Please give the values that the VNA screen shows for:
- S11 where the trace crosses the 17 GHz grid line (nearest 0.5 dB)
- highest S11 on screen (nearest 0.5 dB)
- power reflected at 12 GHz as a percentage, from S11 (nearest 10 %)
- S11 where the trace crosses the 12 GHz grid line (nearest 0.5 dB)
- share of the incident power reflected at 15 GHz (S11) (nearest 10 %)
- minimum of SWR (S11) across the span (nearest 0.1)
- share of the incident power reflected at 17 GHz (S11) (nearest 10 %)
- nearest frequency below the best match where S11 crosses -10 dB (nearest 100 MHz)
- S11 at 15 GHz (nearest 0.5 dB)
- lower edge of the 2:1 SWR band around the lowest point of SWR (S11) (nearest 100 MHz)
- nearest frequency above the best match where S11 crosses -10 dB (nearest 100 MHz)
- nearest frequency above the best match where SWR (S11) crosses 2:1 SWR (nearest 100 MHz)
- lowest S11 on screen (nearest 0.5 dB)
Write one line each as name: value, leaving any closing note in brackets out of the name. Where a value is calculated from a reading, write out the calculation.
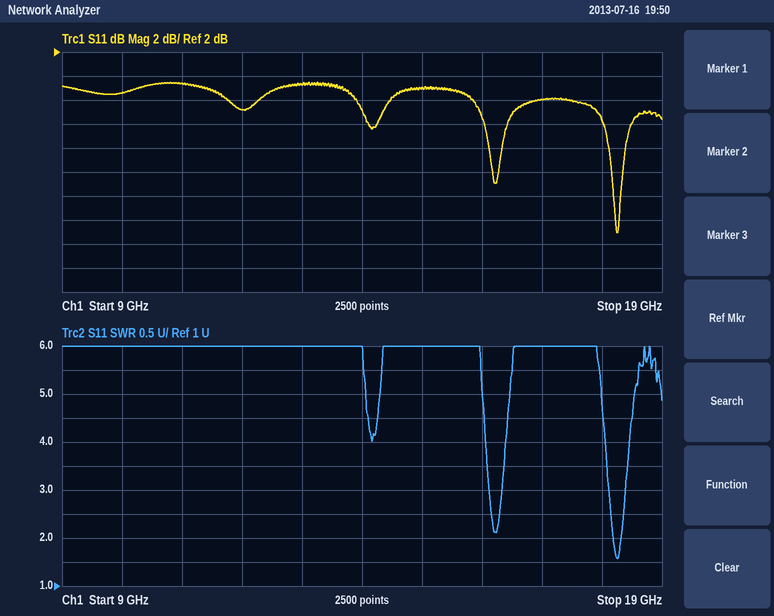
S11 where the trace crosses the 17 GHz grid line: -2.0 dB
highest S11 on screen: -0.5 dB
power reflected at 12 GHz as a percentage, from S11: 10^(-3/10) ≈ 50 %
S11 where the trace crosses the 12 GHz grid line: -3.0 dB
share of the incident power reflected at 15 GHz (S11): 10^(-1/10) ≈ 79.4 %, so 80 % to the nearest 10 %
minimum of SWR (S11) across the span: 1.6
share of the incident power reflected at 17 GHz (S11): 10^(-2/10) ≈ 63.1 %, so 60 % to the nearest 10 %
nearest frequency below the best match where S11 crosses -10 dB: 18.2 GHz
S11 at 15 GHz: -1.0 dB
lower edge of the 2:1 SWR band around the lowest point of SWR (S11): 18.2 GHz
nearest frequency above the best match where S11 crosses -10 dB: 18.3 GHz
nearest frequency above the best match where SWR (S11) crosses 2:1 SWR: 18.3 GHz
lowest S11 on screen: -13.0 dB
